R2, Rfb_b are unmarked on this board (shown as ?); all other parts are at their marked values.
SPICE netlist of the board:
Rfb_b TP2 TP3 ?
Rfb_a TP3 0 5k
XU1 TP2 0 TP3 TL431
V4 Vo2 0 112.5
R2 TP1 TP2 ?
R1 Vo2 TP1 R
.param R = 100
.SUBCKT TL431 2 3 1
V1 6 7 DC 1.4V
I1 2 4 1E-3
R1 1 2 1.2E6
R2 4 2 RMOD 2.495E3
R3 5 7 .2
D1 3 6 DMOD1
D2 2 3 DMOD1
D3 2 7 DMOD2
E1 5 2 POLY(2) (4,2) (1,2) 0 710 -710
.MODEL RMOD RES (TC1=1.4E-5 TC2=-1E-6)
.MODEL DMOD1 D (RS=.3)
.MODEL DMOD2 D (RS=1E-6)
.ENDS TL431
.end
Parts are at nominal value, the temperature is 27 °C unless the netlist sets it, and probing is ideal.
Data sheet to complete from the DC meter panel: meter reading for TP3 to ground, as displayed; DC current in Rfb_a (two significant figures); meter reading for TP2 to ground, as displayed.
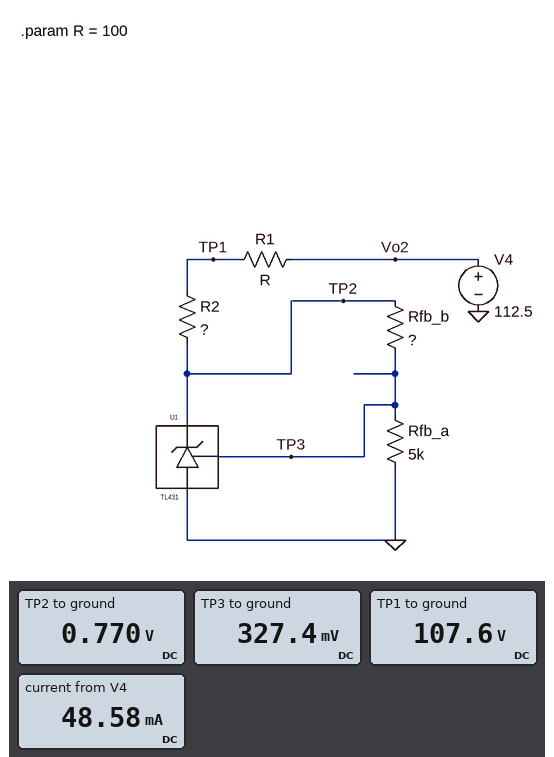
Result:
327.4 mV
65 µA
0.770 V
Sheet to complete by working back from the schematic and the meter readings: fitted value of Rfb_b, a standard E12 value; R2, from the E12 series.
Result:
6.8 kΩ
2.2 kΩ
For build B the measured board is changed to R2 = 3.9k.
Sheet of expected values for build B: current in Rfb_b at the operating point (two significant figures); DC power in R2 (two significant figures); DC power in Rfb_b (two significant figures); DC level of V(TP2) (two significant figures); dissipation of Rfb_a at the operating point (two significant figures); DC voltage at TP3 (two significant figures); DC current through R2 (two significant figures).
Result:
63 µA
3.0 W
27 µW
750 mV
20 µW
320 mV
28 mA
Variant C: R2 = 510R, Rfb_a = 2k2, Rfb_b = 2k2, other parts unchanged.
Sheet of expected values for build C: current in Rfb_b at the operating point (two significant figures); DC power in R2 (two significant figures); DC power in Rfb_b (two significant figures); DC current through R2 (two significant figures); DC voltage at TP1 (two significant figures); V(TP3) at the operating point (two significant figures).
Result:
190 µA
17 W
81 µW
180 mA
94 V
420 mV
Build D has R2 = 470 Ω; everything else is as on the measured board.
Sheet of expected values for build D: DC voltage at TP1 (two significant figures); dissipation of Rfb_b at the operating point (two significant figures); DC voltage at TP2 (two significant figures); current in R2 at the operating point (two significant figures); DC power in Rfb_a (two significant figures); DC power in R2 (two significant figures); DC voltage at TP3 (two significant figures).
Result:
93 V
35 µW
850 mV
200 mA
26 µW
18 W
360 mV
